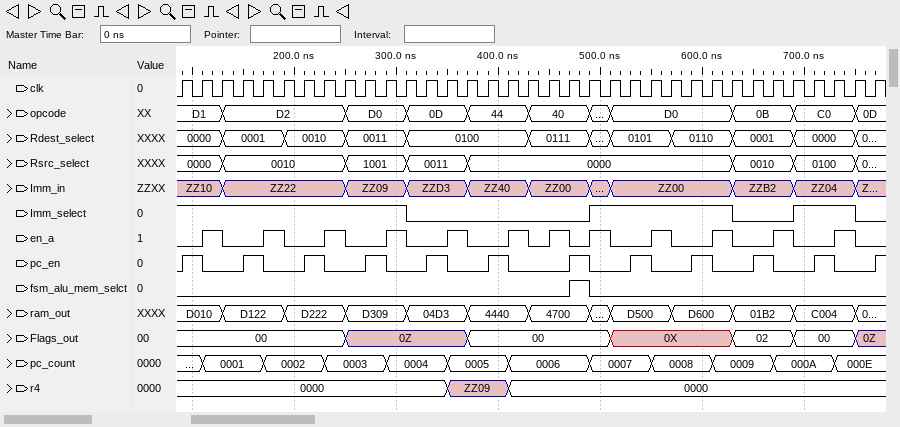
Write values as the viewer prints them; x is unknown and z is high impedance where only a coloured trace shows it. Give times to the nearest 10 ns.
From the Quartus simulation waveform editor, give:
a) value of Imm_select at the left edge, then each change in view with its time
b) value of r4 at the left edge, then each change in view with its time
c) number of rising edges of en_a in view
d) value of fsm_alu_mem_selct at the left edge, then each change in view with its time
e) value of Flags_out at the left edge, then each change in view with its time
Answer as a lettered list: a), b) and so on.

a) 1, 0 at 310 ns, 1 at 490 ns, 0 at 630 ns, 1 at 690 ns, 0 at 750 ns
b) 0000, ZZ09 at 350 ns, 0000 at 410 ns
c) 12
d) 0, 1 at 470 ns, 0 at 490 ns
e) 00, 0Z at 250 ns, 00 at 370 ns, 0X at 510 ns, 02 at 630 ns, 00 at 690 ns, 0Z at 750 ns
